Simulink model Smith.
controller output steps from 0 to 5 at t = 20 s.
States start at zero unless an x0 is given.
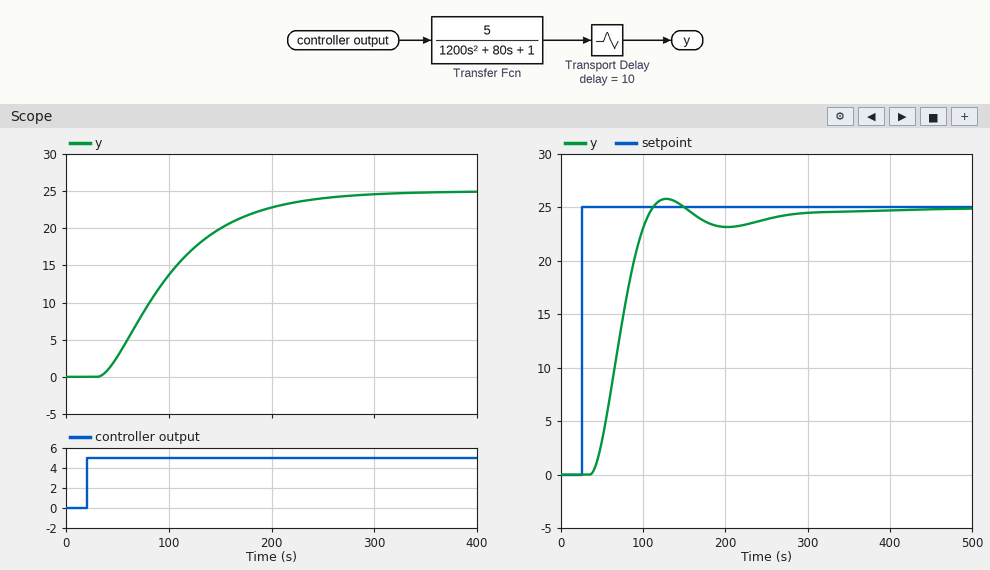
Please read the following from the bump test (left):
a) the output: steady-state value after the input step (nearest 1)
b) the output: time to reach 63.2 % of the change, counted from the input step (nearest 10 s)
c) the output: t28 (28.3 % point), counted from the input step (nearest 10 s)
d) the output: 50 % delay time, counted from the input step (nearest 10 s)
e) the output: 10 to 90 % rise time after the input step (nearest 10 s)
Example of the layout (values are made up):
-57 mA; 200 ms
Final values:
25; 90 s; 50 s; 70 s; 140 s
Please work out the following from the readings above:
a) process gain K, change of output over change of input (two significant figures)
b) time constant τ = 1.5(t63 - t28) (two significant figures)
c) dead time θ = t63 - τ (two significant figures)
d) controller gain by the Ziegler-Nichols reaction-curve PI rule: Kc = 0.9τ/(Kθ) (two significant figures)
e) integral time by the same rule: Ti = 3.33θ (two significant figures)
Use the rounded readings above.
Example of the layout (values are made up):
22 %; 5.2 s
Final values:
5.0; 60 s; 30 s; 0.36; 100 s
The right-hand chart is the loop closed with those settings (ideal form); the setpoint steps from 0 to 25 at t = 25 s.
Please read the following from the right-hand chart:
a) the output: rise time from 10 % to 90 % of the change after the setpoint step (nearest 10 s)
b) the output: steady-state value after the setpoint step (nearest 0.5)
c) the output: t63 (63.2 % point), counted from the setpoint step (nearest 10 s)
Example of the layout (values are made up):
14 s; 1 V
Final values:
50 s; 25.0; 50 s
